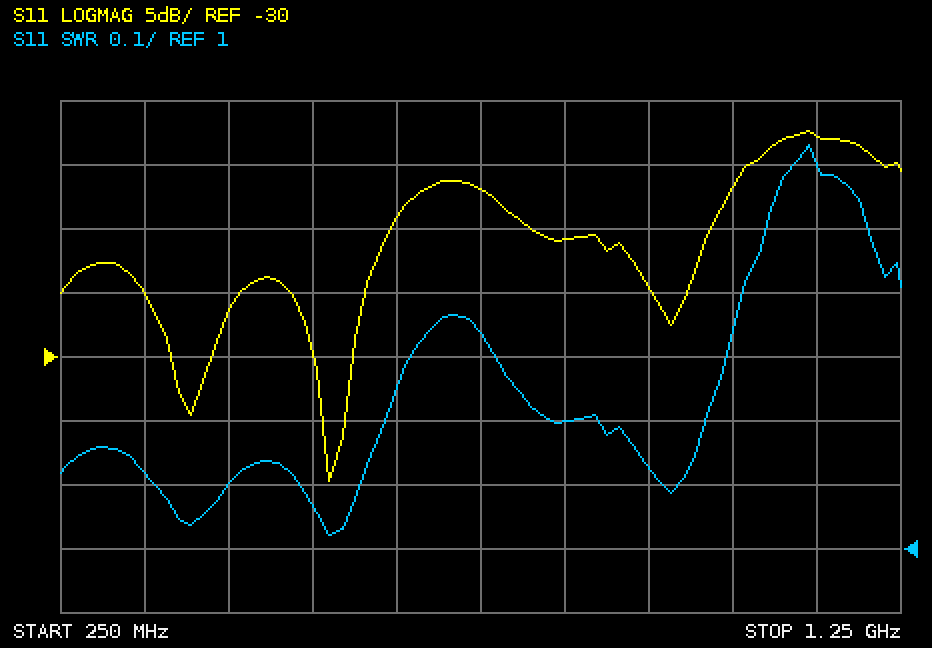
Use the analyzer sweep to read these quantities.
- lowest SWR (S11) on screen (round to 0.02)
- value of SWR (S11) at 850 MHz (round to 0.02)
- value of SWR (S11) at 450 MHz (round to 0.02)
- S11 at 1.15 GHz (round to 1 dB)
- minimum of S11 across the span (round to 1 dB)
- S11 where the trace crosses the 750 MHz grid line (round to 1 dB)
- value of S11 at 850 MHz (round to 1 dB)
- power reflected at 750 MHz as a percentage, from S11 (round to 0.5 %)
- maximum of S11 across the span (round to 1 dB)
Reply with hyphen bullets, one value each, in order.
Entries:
- 1.02
- 1.20
- 1.10
- -13 dB
- -40 dB
- -17 dB
- -21 dB
- 2.0 %
- -12 dB
